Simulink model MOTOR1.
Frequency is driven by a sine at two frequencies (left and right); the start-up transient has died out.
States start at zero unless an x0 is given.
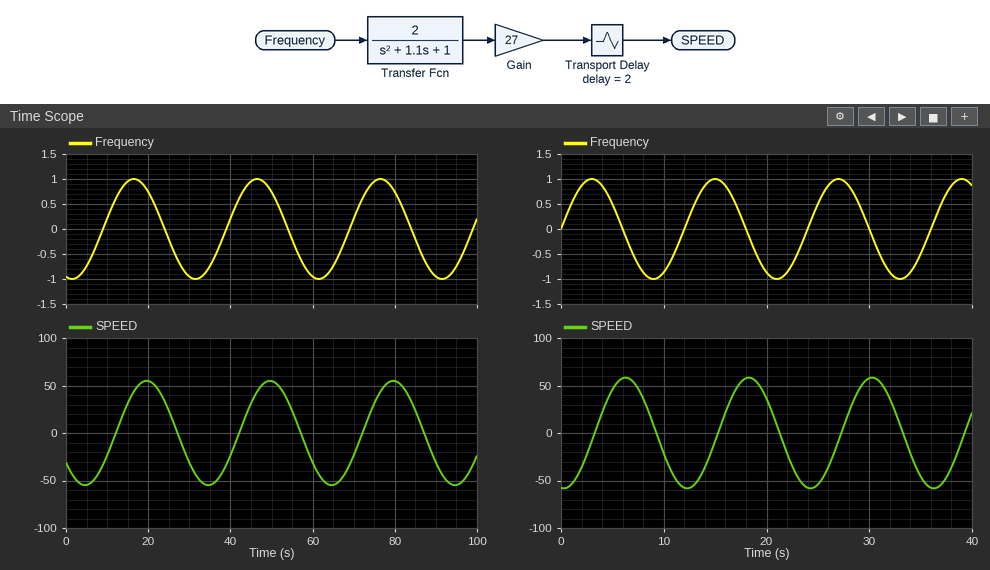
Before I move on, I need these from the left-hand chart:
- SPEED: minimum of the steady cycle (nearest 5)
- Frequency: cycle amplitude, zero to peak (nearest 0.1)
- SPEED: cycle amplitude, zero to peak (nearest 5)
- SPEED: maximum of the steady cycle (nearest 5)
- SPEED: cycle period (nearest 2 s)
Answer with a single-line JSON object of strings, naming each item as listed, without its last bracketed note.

{"SPEED: minimum of the steady cycle": "-55", "Frequency: cycle amplitude, zero to peak": "1.0", "SPEED: cycle amplitude, zero to peak": "55", "SPEED: maximum of the steady cycle": "55", "SPEED: cycle period": "30 s"}
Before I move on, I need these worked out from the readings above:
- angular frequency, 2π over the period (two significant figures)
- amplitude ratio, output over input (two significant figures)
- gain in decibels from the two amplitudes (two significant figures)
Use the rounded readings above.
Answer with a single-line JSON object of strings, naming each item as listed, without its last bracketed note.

{"angular frequency, 2π over the period": "0.21 rad/s", "amplitude ratio, output over input": "55", "gain in decibels from the two amplitudes": "35 dB"}
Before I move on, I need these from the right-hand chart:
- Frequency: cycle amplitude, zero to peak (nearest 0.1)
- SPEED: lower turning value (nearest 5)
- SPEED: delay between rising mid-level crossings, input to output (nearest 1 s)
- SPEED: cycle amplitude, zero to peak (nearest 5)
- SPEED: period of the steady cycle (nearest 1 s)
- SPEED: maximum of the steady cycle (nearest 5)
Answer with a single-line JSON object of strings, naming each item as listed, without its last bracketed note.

{"Frequency: cycle amplitude, zero to peak": "1.0", "SPEED: lower turning value": "-60", "SPEED: delay between rising mid-level crossings, input to output": "3 s", "SPEED: cycle amplitude, zero to peak": "60", "SPEED: period of the steady cycle": "12 s", "SPEED: maximum of the steady cycle": "60"}
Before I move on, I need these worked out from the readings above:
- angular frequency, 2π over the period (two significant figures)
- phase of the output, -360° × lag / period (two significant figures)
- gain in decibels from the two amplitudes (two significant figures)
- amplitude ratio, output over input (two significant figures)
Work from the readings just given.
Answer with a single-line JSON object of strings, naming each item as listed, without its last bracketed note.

{"angular frequency, 2π over the period": "0.52 rad/s", "phase of the output, -360° × lag / period": "-90°", "gain in decibels from the two amplitudes": "36 dB", "amplitude ratio, output over input": "60"}
